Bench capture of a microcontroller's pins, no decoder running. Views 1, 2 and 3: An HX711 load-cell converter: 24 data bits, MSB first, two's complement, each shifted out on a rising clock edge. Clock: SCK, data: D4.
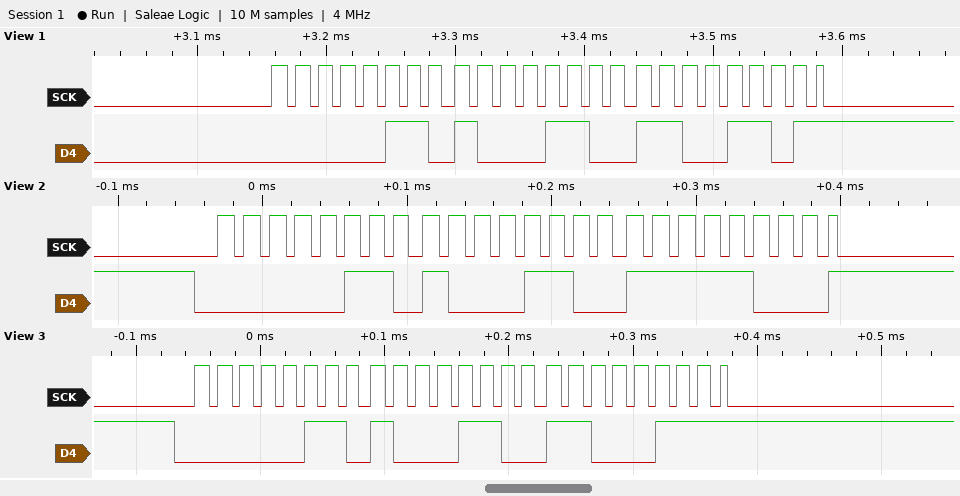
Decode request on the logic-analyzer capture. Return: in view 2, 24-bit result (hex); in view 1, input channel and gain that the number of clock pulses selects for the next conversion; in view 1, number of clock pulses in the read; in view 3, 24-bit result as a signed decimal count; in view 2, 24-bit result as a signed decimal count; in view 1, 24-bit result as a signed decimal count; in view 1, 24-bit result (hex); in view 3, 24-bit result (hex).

0x068CF8
channel A, gain 128
25
429255
429304
429261
0x068CCD
0x068CC7
